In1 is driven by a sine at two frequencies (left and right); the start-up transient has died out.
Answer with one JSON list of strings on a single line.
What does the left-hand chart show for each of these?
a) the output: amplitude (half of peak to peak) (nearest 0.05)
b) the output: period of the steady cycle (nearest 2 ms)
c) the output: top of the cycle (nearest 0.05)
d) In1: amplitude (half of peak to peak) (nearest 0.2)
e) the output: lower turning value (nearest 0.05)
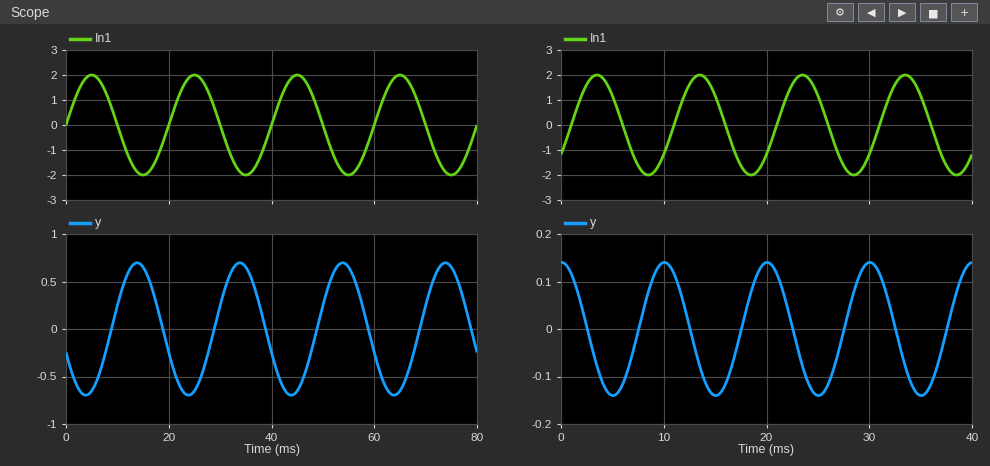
["0.70", "20 ms", "0.70", "2.0", "-0.70"]
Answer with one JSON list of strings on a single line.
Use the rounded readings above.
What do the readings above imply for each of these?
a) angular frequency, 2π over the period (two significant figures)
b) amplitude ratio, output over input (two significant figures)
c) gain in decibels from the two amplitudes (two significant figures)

["0.31 rad/ms", "0.35", "-9.1 dB"]
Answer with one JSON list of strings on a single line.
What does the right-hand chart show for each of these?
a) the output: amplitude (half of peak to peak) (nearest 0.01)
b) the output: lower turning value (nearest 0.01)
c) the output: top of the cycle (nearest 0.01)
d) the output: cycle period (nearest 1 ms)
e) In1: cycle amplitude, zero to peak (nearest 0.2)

["0.14", "-0.14", "0.14", "10 ms", "2.0"]
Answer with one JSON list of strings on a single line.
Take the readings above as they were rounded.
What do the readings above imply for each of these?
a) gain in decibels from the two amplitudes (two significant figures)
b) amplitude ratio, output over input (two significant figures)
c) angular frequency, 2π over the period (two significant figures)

["-23 dB", "0.070", "0.63 rad/ms"]
